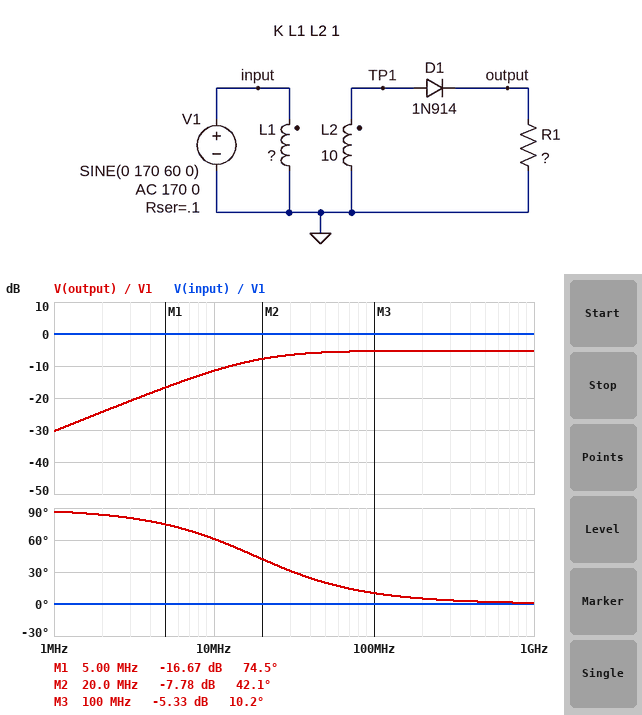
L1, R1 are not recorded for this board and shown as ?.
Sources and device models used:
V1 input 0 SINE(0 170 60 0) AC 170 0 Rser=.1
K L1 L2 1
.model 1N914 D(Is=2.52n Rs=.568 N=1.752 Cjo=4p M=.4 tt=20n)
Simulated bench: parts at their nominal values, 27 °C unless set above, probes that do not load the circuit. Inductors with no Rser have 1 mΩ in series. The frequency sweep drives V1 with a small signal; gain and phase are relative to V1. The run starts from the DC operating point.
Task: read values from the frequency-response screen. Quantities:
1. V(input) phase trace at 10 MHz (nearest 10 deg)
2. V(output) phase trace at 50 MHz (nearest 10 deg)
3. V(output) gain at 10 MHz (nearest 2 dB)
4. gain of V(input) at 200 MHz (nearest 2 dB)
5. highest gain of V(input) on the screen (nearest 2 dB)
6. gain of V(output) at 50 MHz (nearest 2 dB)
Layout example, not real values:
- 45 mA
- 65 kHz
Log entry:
- 0 deg
- 20 deg
- -12 dB
- 0 dB
- 0 dB
- -6 dB
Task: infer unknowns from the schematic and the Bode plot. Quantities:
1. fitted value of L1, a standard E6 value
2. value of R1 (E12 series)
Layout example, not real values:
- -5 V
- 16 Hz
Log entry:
- 33 H
- 2.2 kΩ
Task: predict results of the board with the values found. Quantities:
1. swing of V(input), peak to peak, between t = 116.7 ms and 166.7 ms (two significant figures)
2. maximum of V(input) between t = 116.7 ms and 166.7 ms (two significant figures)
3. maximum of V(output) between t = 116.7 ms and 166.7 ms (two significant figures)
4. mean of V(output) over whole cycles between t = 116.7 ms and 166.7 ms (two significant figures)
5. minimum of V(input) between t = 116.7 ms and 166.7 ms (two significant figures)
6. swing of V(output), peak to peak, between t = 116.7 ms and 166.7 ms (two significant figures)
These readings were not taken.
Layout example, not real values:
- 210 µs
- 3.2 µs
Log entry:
- 340 V
- 170 V
- 93 V
- 29 V
- -170 V
- 93 V
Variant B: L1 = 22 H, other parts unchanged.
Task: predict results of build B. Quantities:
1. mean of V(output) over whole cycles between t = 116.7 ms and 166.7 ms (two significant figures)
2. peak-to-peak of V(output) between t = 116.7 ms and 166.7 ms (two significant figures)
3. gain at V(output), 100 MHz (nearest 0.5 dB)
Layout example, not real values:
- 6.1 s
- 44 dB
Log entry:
- 36 V
- 110 V
- -3.5 dB
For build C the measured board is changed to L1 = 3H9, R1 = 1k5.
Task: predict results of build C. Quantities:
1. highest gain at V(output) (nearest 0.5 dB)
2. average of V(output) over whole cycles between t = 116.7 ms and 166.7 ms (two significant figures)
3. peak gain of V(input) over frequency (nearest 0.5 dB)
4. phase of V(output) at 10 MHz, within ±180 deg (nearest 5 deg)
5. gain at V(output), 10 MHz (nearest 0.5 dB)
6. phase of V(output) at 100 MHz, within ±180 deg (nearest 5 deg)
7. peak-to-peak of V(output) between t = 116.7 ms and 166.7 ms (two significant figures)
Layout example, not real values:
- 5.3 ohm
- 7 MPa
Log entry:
- 4.0 dB
- 86 V
- 0 dB
- 70 deg
- -5.0 dB
- 15 deg
- 270 V
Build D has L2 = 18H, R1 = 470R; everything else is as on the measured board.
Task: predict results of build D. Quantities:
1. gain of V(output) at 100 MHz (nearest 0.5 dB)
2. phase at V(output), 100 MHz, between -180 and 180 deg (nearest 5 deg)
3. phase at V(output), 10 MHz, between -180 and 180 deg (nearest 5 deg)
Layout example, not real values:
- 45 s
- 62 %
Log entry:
- -5.0 dB
- 40 deg
- 85 deg
